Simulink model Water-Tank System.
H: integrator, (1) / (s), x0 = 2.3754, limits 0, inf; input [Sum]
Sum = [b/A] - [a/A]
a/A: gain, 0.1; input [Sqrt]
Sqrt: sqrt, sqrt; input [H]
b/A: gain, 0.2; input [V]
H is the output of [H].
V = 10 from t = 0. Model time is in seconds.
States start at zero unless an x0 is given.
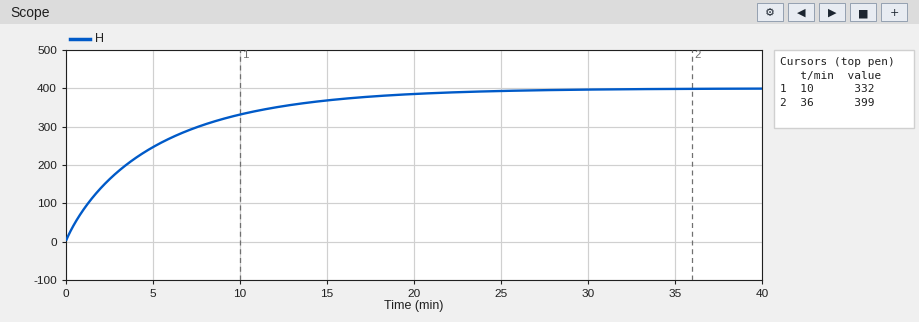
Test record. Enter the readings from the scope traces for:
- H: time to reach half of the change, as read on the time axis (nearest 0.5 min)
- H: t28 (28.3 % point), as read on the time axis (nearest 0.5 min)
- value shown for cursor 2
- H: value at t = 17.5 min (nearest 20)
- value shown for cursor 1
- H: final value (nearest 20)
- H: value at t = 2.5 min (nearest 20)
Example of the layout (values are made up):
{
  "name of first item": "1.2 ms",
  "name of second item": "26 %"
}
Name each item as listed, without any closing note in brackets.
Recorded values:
{
  "H: time to reach half of the change, as read on the time axis": "3.5 min",
  "H: t28 (28.3 % point), as read on the time axis": "1.5 min",
  "value shown for cursor 2": "399",
  "H: value at t = 17.5 min": "380",
  "value shown for cursor 1": "332",
  "H: final value": "400",
  "H: value at t = 2.5 min": "160"
}
